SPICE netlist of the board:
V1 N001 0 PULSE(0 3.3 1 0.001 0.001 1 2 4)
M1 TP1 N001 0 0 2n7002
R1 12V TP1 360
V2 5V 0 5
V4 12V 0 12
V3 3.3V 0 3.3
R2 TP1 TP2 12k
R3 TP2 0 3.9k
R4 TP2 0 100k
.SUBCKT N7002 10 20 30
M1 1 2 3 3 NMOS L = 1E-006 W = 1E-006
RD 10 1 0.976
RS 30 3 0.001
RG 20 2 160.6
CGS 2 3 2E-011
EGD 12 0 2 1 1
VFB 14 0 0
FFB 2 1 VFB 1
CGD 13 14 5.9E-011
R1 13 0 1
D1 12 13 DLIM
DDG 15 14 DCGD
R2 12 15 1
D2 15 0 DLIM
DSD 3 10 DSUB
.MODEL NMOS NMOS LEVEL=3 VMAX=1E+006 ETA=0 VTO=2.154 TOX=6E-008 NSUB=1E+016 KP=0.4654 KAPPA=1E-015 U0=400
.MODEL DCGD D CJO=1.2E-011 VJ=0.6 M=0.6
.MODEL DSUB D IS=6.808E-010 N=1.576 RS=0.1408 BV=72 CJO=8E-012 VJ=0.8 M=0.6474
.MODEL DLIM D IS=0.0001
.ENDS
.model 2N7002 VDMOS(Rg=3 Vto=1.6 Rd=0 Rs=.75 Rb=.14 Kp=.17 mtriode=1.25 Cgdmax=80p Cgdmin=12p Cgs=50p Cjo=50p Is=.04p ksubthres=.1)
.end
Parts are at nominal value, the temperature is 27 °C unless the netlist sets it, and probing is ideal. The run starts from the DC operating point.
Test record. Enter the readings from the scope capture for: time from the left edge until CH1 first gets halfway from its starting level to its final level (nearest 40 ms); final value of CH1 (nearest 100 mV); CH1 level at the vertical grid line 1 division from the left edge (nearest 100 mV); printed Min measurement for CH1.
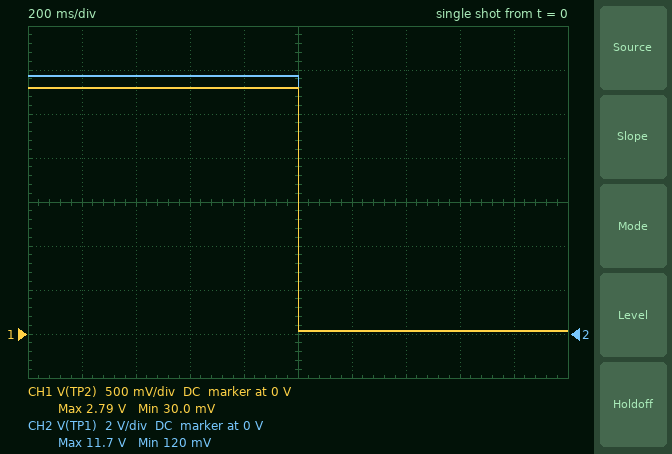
1.00 s
0 V
2.8 V
30.0 mV
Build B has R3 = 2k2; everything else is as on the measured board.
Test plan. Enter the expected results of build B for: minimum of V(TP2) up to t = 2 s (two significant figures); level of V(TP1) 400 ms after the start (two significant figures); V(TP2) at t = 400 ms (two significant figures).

18 mV
12 V
1.8 V
